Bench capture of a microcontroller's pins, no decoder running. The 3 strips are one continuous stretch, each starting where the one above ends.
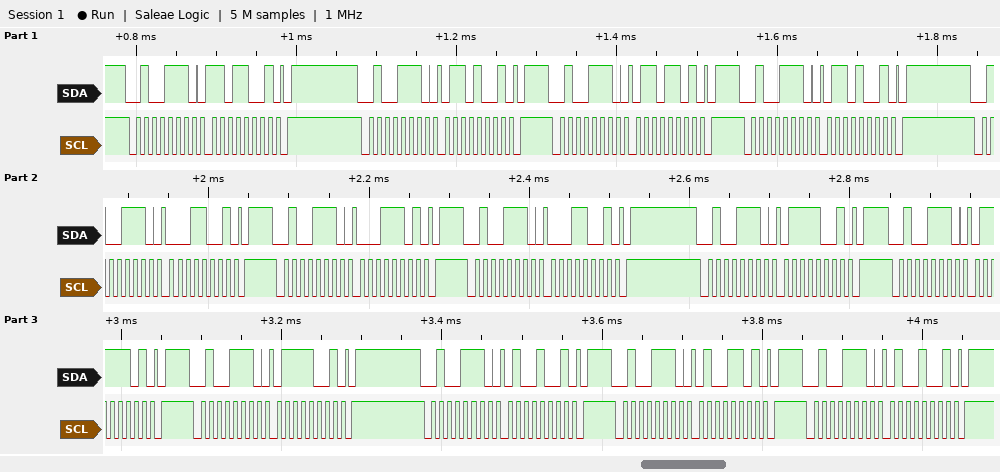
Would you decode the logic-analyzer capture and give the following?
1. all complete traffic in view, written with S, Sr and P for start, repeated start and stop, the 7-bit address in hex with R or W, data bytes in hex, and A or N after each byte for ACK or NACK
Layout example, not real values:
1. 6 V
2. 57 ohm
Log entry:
1. S 27W A D9 A P S 27W A 69 A P S 27W A 6D A P S 27W A 69 A P S 27W A 19 A P S 27W A 1D A P S 27W A 19 A P S 27W A 79 A P S 27W A 7D A P S 27W A 79 A P S 27W A 49 A P S 27W A 4D A P S 27W A 49 A P
